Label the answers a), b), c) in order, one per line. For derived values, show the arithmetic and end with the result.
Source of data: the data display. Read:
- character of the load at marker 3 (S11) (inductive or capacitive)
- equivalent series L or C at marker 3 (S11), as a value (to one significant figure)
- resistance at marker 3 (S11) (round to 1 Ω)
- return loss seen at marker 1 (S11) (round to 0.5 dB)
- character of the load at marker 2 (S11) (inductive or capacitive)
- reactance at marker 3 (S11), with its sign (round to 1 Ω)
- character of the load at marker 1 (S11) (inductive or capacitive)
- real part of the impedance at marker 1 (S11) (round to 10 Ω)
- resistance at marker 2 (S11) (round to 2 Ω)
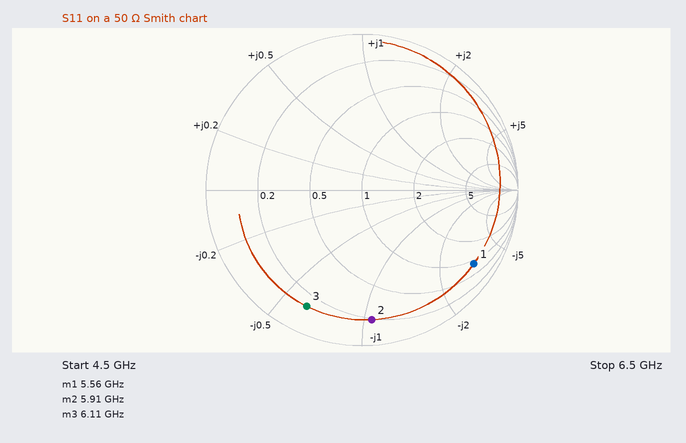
a) capacitive
b) C = 1/(2π × 6.11 GHz × 31 Ω) ≈ 840 fF, so 800 fF to one significant figure
c) 7 Ω
d) 1.5 dB
e) capacitive
f) -31 Ω
g) capacitive
h) 40 Ω
i) 10 Ω
